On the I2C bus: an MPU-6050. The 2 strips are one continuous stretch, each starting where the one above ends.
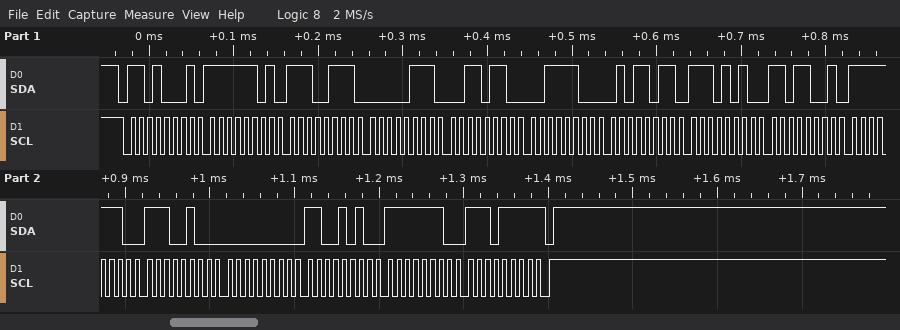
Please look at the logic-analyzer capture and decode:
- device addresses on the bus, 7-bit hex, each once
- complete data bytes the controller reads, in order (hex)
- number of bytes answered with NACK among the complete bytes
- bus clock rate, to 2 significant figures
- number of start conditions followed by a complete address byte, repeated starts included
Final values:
0x68
FD E7 07 36 3C 5B EA D9 FE E4 00 CA FE EF
1
100 kHz
1
